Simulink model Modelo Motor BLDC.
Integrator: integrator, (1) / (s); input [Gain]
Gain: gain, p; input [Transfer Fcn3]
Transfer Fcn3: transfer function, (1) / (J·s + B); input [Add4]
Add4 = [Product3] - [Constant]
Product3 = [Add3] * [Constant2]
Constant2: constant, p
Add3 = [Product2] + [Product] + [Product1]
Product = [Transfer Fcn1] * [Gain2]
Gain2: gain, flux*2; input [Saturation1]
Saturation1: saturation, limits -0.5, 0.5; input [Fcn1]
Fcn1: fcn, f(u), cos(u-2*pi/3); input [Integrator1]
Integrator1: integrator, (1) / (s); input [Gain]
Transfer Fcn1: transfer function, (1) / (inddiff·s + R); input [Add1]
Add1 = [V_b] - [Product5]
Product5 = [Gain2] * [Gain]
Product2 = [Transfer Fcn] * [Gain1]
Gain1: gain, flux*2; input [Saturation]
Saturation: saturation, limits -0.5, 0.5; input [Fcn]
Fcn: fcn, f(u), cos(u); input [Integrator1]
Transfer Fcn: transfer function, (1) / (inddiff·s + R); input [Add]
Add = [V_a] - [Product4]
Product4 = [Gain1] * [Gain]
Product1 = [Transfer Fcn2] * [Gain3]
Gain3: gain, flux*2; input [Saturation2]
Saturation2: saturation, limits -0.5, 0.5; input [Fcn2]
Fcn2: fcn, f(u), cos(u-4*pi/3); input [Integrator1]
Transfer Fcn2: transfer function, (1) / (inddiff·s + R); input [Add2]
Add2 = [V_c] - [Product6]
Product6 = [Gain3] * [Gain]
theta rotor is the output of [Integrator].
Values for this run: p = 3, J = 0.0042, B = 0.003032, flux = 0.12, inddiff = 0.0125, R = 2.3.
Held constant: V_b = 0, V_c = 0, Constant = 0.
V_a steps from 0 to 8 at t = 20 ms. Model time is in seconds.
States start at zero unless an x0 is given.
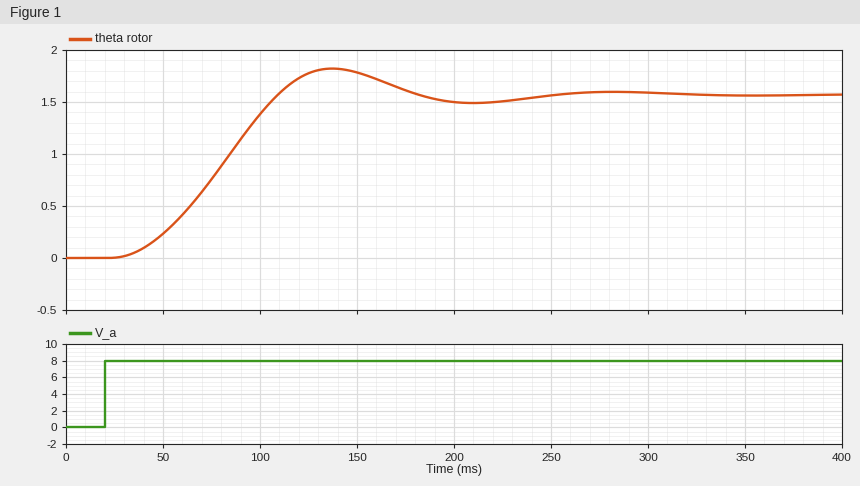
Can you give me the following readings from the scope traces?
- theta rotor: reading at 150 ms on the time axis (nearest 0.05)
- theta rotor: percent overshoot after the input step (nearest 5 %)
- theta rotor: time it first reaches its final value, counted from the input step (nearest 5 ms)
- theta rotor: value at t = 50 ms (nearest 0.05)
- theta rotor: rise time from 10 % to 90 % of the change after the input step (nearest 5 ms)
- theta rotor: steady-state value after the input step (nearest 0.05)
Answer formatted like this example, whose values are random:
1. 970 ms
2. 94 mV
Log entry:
1. 1.80
2. 15 %
3. 90 ms
4. 0.25
5. 55 ms
6. 1.55
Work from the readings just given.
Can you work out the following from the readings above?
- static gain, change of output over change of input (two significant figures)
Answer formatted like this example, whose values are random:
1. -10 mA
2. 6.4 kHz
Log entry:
1. 0.19
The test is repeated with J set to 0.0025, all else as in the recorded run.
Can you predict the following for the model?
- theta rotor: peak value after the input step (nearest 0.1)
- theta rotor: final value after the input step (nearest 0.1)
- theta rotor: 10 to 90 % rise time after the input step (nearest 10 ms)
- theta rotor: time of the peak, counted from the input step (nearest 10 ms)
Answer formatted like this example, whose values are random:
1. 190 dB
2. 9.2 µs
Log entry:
1. 1.7
2. 1.6
3. 50 ms
4. 100 ms
